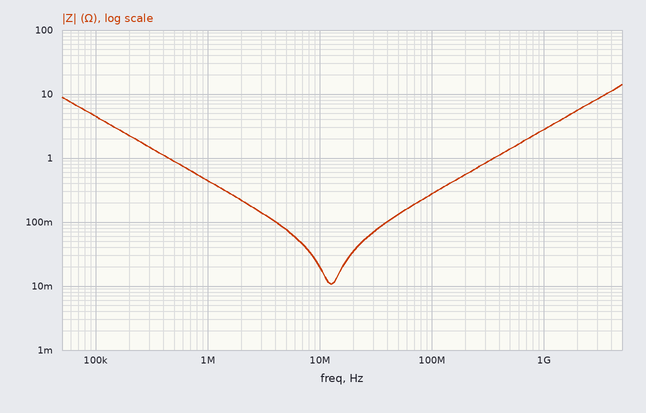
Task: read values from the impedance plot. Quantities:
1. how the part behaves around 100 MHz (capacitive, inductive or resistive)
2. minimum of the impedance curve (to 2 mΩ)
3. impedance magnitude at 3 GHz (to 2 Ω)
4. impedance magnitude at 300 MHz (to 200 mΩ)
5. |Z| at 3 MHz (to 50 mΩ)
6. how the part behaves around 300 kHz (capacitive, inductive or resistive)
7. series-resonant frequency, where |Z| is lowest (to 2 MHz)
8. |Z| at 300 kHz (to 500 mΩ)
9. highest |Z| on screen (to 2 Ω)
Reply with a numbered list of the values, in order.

1. inductive
2. 10 mΩ
3. 8 Ω
4. 800 mΩ
5. 150 mΩ
6. capacitive
7. 12 MHz
8. 1.5 Ω
9. 14 Ω
